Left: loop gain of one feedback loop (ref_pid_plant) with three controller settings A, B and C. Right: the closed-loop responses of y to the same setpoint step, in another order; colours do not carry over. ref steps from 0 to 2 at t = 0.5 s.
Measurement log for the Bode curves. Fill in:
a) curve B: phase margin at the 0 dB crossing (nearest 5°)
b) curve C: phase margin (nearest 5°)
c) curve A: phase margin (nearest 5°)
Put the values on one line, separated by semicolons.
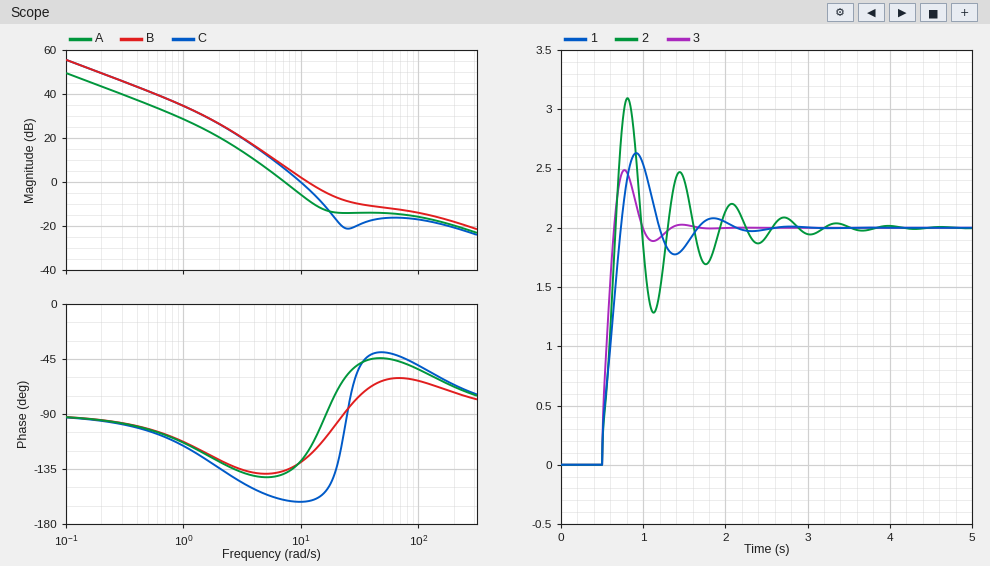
55°; 20°; 40°
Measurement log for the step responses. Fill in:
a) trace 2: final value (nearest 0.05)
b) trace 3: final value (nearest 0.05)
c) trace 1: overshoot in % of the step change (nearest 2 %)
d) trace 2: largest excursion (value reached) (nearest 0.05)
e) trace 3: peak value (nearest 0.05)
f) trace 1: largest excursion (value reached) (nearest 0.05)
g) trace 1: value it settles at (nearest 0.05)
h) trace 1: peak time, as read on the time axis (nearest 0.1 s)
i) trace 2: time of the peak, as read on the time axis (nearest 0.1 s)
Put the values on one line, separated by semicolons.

2.00; 2.00; 32 %; 3.10; 2.50; 2.65; 2.00; 0.9 s; 0.8 s
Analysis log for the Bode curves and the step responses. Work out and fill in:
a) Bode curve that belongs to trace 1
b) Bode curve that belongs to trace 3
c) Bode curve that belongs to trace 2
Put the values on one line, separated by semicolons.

A; B; C
